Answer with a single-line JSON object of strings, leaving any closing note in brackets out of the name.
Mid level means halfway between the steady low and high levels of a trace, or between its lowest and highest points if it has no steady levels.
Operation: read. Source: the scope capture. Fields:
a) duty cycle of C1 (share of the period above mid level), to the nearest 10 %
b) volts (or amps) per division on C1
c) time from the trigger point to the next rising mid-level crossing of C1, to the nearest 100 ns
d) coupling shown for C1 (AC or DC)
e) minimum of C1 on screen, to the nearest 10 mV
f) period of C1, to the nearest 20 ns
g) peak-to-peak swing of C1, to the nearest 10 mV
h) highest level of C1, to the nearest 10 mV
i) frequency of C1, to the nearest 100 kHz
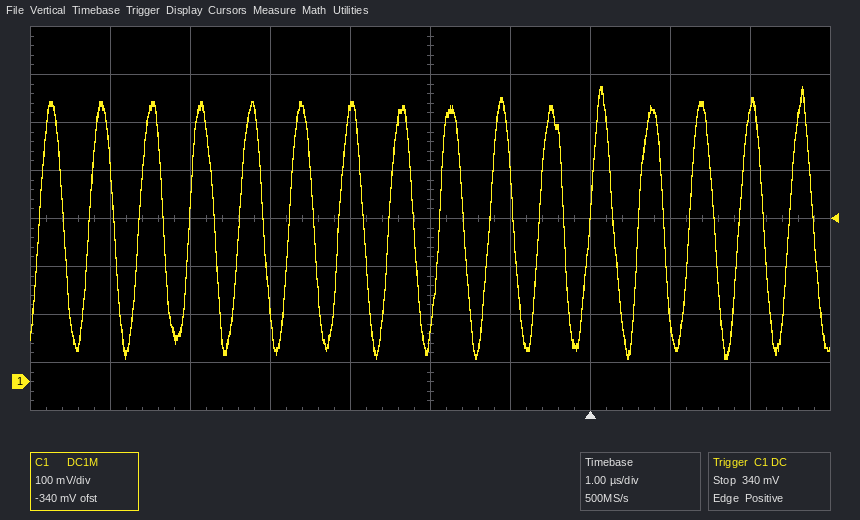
{"duty cycle of C1 (share of the period above mid level), to the nearest 10 %": "50 %", "volts (or amps) per division on C1": "100 mV", "time from the trigger point to the next rising mid-level crossing of C1, to the nearest 100 ns": "600 ns", "coupling shown for C1": "DC", "minimum of C1 on screen, to the nearest 10 mV": "50 mV", "period of C1, to the nearest 20 ns": "620 ns", "peak-to-peak swing of C1, to the nearest 10 mV": "570 mV", "highest level of C1, to the nearest 10 mV": "620 mV", "frequency of C1, to the nearest 100 kHz": "1.6 MHz"}
